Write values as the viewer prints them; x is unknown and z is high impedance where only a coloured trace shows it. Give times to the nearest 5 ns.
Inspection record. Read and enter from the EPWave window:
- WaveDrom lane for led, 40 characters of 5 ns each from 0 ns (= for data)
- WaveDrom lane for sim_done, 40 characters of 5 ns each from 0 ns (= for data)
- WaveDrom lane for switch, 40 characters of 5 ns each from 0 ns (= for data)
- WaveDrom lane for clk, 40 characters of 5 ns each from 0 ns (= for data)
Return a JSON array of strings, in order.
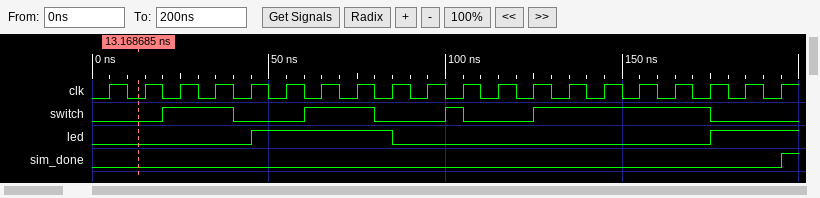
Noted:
["{name: 'led', wave: '0........1.......0.................1....'}", "{name: 'sim_done', wave: '0......................................1'}", "{name: 'switch', wave: '0...1...0...1...0...10...1.........0....'}", "{name: 'clk', wave: '0101010101010101010101010101010101010101'}"]
